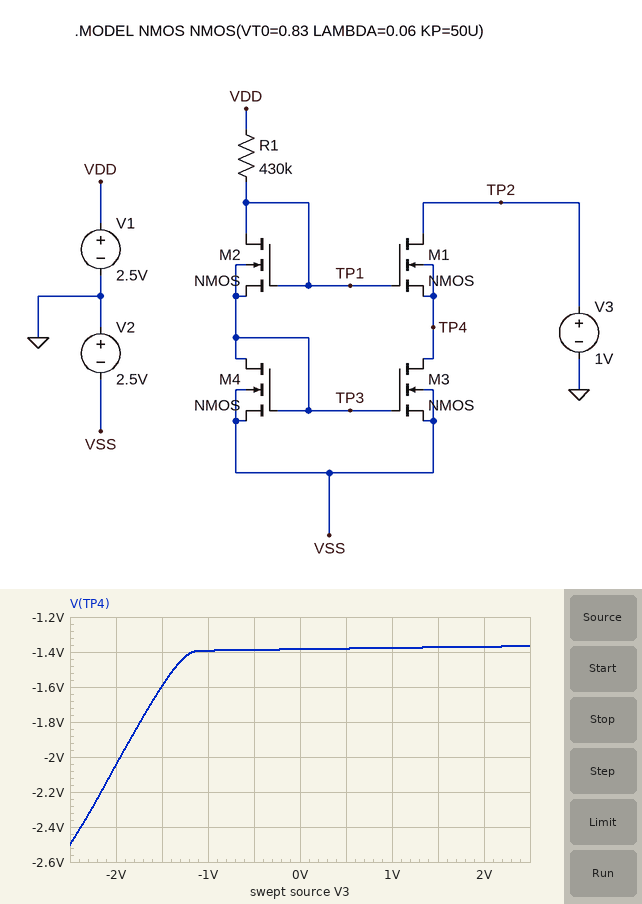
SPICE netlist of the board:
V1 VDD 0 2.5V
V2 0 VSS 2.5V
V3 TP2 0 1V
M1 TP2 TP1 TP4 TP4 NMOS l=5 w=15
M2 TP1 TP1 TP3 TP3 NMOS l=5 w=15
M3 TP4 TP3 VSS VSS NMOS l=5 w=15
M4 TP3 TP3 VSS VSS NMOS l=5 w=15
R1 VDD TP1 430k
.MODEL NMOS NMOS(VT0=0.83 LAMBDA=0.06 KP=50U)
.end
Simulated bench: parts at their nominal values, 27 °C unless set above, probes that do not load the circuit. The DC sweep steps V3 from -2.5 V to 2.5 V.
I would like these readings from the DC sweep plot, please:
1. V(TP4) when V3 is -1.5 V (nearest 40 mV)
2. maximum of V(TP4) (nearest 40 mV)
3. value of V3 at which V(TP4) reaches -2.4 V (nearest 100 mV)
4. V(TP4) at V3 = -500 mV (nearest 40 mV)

-1.60 V
-1.36 V
-2.4 V
-1.40 V
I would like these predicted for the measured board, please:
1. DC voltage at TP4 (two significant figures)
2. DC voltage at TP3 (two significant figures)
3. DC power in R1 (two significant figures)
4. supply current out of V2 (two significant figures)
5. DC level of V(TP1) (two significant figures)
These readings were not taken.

-1.4 V
-1.4 V
18 µW
13 µA
-270 mV
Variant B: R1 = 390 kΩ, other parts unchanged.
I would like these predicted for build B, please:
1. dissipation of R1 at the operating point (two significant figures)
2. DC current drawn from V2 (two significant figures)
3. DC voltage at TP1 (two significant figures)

19 µW
14 µA
-250 mV
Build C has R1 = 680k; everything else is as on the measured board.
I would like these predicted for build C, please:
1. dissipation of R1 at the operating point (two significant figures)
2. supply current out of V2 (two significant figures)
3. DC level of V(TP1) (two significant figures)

12 µW
8.5 µA
-380 mV
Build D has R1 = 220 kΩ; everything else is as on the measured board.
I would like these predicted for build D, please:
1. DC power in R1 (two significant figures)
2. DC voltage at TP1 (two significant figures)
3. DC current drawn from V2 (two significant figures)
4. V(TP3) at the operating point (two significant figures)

30 µW
-77 mV
23 µA
-1.3 V
